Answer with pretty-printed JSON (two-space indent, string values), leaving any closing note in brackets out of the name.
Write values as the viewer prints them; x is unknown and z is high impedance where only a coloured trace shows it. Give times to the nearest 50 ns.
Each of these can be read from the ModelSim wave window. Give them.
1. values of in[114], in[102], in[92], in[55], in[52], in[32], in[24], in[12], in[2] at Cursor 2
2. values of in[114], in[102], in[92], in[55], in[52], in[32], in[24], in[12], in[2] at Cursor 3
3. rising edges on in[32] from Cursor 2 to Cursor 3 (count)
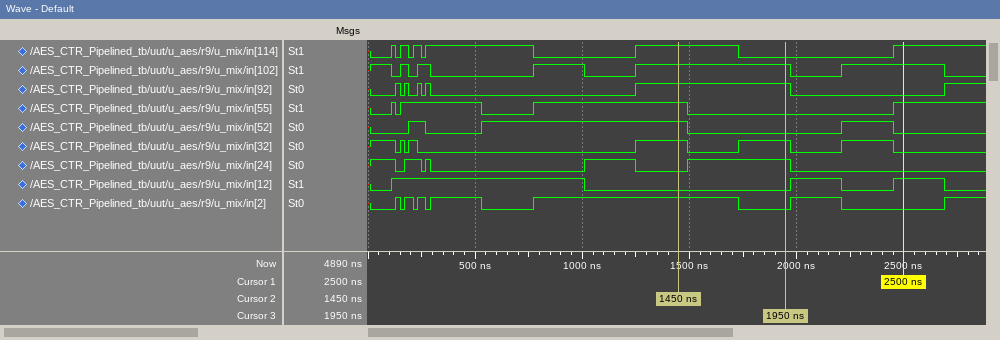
{
  "values of in[114], in[102], in[92], in[55], in[52], in[32], in[24], in[12], in[2] at Cursor 2": "in[114]=1, in[102]=1, in[92]=1, in[55]=1, in[52]=1, in[32]=1, in[24]=0, in[12]=0, in[2]=1",
  "values of in[114], in[102], in[92], in[55], in[52], in[32], in[24], in[12], in[2] at Cursor 3": "in[114]=0, in[102]=1, in[92]=1, in[55]=0, in[52]=0, in[32]=1, in[24]=1, in[12]=0, in[2]=0",
  "rising edges on in[32] from Cursor 2 to Cursor 3": "1"
}
